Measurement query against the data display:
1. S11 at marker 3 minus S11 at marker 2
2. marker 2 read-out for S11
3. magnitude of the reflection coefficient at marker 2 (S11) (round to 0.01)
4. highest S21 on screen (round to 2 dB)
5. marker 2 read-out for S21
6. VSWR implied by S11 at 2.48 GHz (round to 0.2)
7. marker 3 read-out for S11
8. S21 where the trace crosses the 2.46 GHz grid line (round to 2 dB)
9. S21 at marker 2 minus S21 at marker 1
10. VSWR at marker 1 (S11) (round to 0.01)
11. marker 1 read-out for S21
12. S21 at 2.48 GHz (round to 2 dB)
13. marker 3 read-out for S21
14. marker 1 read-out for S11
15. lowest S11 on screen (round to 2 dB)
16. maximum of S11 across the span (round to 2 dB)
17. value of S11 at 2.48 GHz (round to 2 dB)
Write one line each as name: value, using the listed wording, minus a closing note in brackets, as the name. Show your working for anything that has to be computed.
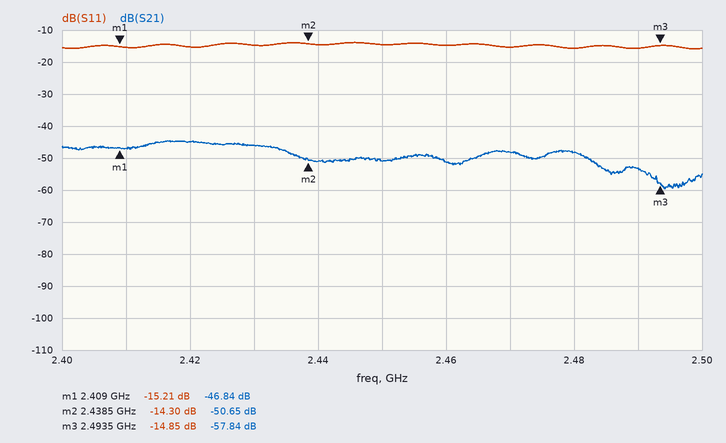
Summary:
S11 at marker 3 minus S11 at marker 2: -14.85 − (-14.3) = -0.55 dB
marker 2 read-out for S11: -14.30 dB
magnitude of the reflection coefficient at marker 2 (S11): 10^(-14.3/20) ≈ 0.19
highest S21 on screen: -44 dB
marker 2 read-out for S21: -50.65 dB
VSWR implied by S11 at 2.48 GHz: |Γ| = 10^(-16/20) = 0.1585; VSWR = (1 + 0.1585)/(1 − 0.1585) ≈ 1.4
marker 3 read-out for S11: -14.85 dB
S21 where the trace crosses the 2.46 GHz grid line: -52 dB
S21 at marker 2 minus S21 at marker 1: -50.65 − (-46.84) = -3.81 dB
VSWR at marker 1 (S11): (1 + 0.1736)/(1 − 0.1736) ≈ 1.42
marker 1 read-out for S21: -46.84 dB
S21 at 2.48 GHz: -48 dB
marker 3 read-out for S21: -57.84 dB
marker 1 read-out for S11: -15.21 dB
lowest S11 on screen: -16 dB
maximum of S11 across the span: -14 dB
value of S11 at 2.48 GHz: -16 dB
